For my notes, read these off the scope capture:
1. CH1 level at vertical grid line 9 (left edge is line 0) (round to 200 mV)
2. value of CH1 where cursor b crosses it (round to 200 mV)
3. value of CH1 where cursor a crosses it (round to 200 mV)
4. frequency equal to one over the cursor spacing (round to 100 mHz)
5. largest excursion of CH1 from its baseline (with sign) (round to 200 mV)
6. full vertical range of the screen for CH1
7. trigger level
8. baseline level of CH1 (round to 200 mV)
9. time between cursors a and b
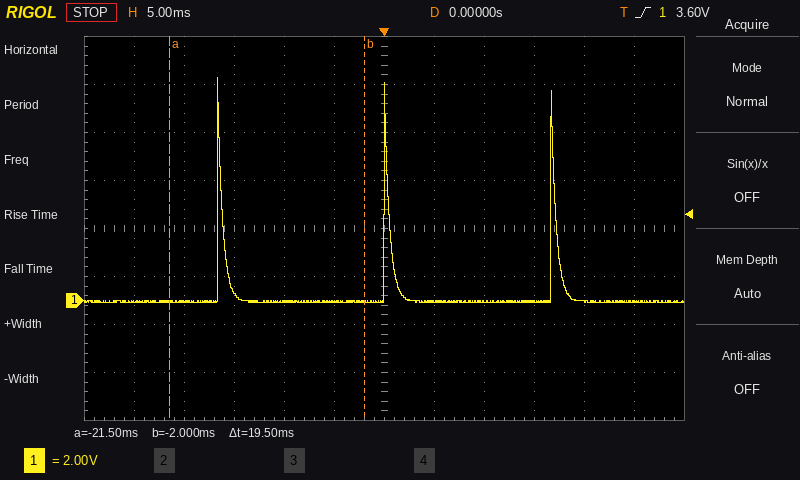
0.0 V
0.0 V
0.0 V
51.3 Hz
+9.4 V
16 V
3.60 V
0.0 V
19.5 ms
